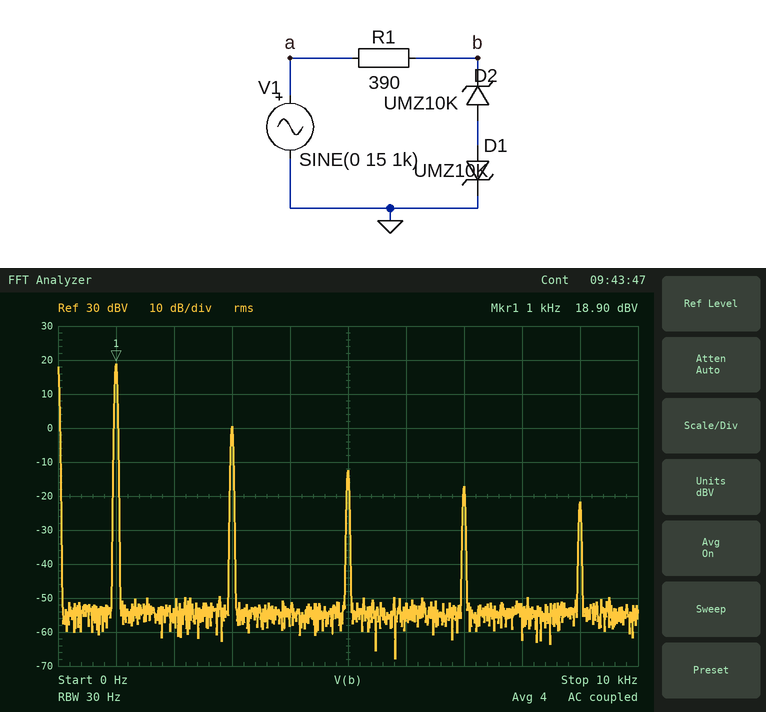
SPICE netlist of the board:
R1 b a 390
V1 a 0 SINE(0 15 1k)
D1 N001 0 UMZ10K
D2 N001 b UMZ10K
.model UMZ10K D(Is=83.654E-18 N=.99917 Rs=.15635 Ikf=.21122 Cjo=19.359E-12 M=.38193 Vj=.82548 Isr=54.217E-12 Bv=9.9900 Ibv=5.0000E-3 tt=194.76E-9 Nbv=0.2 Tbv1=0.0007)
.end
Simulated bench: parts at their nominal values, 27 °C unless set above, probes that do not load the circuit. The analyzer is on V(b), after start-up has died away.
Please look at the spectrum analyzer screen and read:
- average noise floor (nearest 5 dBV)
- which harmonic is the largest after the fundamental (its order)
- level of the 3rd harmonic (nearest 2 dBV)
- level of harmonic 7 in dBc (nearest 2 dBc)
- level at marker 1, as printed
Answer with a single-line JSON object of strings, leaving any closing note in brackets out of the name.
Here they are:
{"average noise floor": "-55 dBV", "which harmonic is the largest after the fundamental": "3", "level of the 3rd harmonic": "0 dBV", "level of harmonic 7 in dBc": "-36 dBc", "level at marker 1, as printed": "18.90 dBV"}
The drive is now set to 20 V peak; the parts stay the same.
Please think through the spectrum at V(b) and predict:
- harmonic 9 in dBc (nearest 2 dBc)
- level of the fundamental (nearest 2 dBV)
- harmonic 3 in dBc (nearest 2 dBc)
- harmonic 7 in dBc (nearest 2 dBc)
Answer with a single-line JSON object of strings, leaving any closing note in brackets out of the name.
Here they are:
{"harmonic 9 in dBc": "-34 dBc", "level of the fundamental": "20 dBV", "harmonic 3 in dBc": "-14 dBc", "harmonic 7 in dBc": "-32 dBc"}
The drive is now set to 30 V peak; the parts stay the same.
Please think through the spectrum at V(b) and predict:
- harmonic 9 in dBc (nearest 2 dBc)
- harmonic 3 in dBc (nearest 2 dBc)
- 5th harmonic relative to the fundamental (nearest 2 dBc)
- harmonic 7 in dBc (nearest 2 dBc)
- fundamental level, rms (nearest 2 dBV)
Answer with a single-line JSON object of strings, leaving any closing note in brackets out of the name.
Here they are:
{"harmonic 9 in dBc": "-48 dBc", "harmonic 3 in dBc": "-12 dBc", "5th harmonic relative to the fundamental": "-20 dBc", "harmonic 7 in dBc": "-30 dBc", "fundamental level, rms": "20 dBV"}
